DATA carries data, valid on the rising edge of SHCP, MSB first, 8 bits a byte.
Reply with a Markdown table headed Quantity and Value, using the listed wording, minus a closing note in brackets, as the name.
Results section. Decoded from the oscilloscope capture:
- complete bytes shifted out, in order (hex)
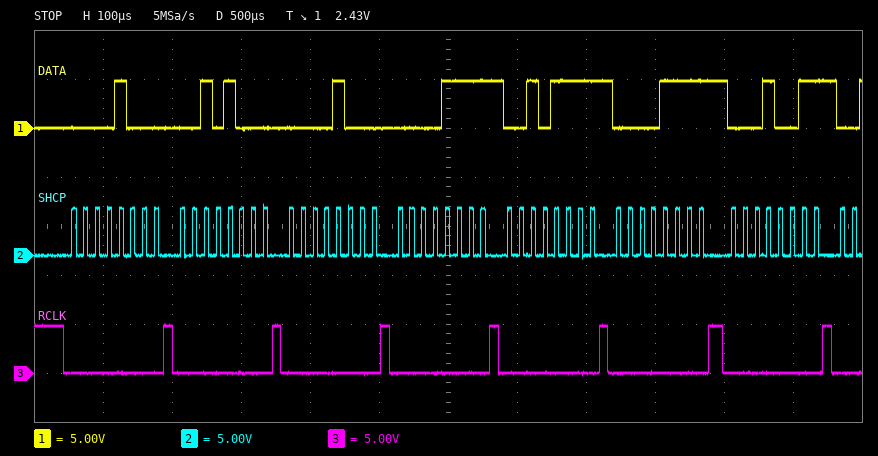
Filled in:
| Quantity | Value |
|---|---|
| complete bytes shifted out, in order | 0x08 0x28 0x08 0x0F 0x2F 0x0F 0x13 |
